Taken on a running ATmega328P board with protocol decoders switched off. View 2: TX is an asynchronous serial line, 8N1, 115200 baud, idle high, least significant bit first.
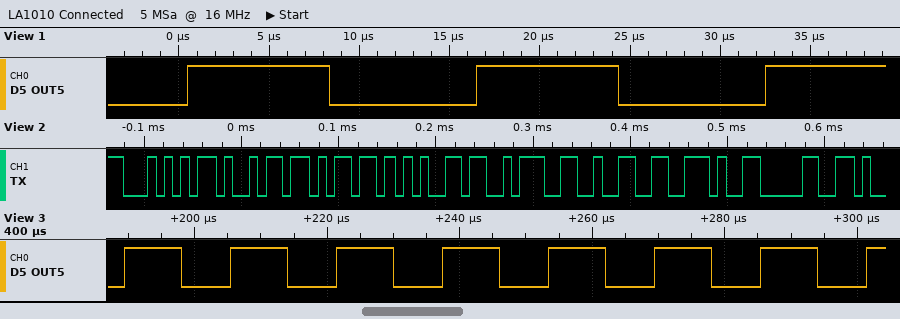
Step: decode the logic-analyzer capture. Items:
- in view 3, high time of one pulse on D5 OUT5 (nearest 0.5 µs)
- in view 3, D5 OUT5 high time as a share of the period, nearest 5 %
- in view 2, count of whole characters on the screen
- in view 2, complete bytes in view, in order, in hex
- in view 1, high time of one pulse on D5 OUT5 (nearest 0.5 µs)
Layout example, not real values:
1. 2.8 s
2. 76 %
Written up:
1. 8.5 µs
2. 55 %
3. 8
4. 54 69 6D 65 3A 32 2E 30
5. 8.0 µs
